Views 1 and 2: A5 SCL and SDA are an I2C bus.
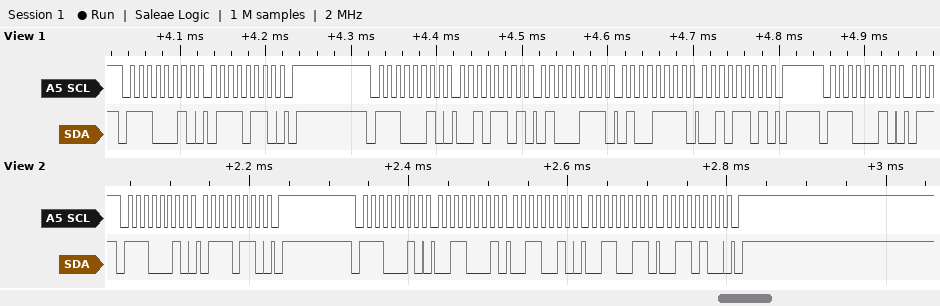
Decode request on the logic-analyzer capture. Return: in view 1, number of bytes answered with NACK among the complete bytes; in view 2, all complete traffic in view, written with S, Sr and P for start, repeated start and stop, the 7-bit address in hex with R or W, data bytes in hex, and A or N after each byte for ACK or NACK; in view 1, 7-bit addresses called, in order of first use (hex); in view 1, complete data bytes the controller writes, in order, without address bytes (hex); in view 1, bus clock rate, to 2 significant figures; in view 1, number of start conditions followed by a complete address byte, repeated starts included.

0
S 71W A 76 A P S 71W A 31 A 32 A 33 A 34 A P
0x71
76 2D 47 4F 2D
100 kHz
3
